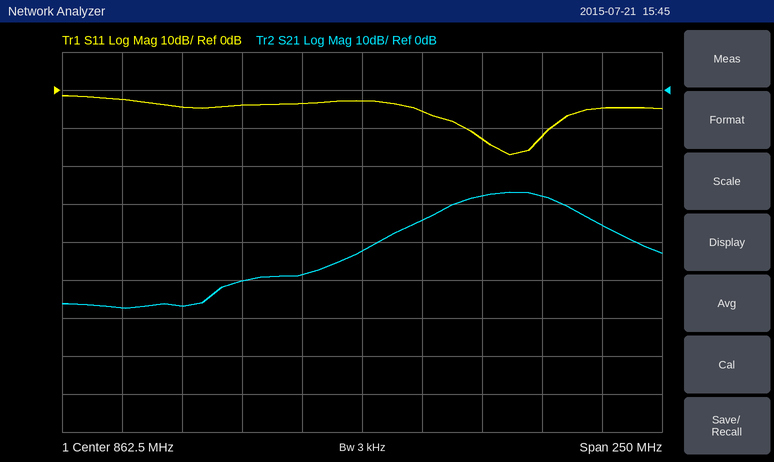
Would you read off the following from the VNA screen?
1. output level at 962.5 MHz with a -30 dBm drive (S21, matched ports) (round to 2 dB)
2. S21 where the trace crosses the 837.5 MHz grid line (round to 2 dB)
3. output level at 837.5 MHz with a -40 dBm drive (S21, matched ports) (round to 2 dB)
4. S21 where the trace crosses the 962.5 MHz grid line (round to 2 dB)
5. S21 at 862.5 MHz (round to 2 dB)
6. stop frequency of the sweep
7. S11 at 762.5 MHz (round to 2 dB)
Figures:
-66 dBm
-48 dB
-88 dBm
-36 dB
-42 dB
987.5 MHz
-2 dB
